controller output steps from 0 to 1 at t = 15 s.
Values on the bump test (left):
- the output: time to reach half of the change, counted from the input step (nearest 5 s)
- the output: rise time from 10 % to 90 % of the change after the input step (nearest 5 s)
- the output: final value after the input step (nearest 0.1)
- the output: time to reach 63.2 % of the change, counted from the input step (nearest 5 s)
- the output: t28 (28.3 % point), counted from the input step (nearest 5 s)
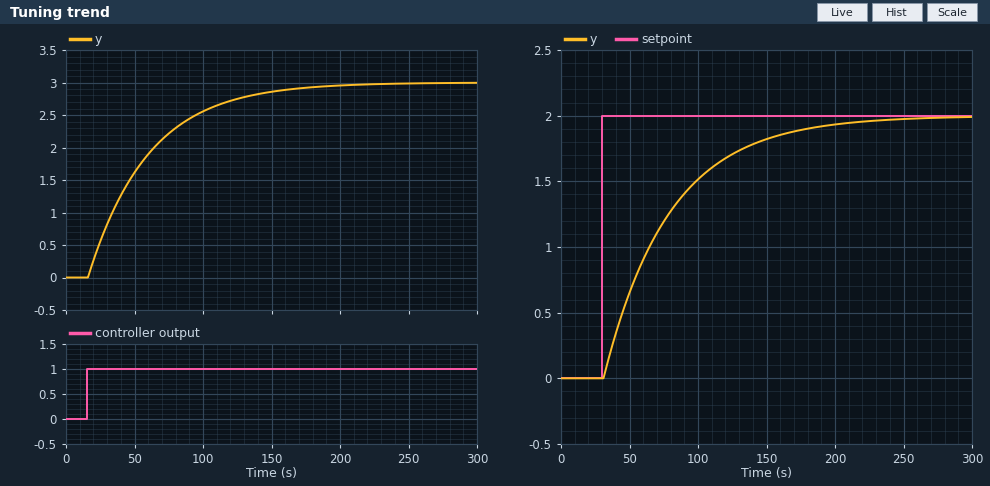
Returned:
30 s
95 s
3.0
45 s
15 s
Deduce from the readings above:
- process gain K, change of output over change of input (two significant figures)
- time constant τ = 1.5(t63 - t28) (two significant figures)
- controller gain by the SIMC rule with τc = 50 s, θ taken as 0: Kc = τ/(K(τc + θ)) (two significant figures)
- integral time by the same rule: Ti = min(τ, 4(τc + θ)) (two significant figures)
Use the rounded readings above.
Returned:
3.0
45 s
0.30
45 s
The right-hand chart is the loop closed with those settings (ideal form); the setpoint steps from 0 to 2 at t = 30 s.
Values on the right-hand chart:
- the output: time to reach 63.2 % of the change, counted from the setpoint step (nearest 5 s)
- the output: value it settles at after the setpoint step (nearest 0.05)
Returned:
50 s
2.00
